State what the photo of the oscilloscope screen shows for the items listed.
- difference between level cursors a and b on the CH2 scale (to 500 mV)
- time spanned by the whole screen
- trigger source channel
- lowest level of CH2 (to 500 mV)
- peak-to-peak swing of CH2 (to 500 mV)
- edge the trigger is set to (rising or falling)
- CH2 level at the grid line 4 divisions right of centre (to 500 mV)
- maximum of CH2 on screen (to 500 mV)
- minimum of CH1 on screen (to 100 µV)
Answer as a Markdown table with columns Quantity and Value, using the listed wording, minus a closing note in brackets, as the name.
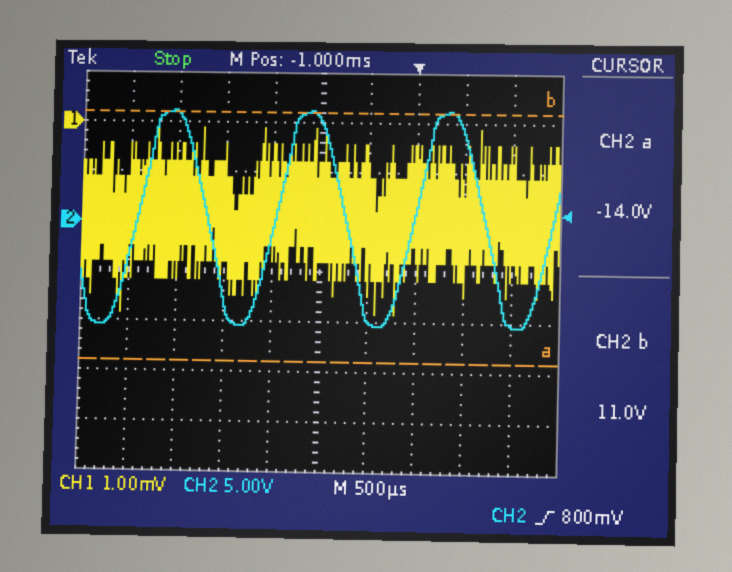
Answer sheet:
| Quantity | Value |
|---|---|
| difference between level cursors a and b on the CH2 scale | 25.0 V |
| time spanned by the whole screen | 5 ms |
| trigger source channel | CH2 |
| lowest level of CH2 | -10.5 V |
| peak-to-peak swing of CH2 | 21.5 V |
| edge the trigger is set to | rising |
| CH2 level at the grid line 4 divisions right of centre | -10.0 V |
| maximum of CH2 on screen | 11.0 V |
| minimum of CH1 on screen | -3.8 mV |
